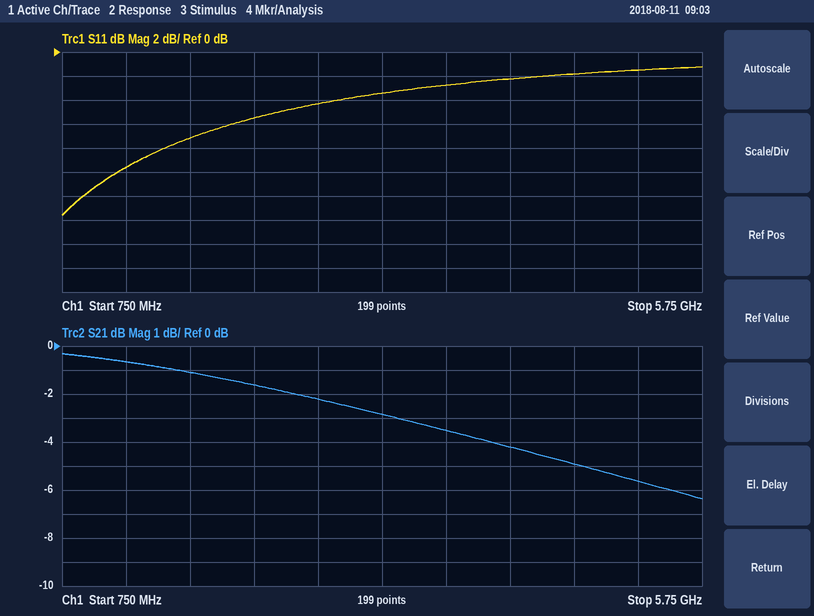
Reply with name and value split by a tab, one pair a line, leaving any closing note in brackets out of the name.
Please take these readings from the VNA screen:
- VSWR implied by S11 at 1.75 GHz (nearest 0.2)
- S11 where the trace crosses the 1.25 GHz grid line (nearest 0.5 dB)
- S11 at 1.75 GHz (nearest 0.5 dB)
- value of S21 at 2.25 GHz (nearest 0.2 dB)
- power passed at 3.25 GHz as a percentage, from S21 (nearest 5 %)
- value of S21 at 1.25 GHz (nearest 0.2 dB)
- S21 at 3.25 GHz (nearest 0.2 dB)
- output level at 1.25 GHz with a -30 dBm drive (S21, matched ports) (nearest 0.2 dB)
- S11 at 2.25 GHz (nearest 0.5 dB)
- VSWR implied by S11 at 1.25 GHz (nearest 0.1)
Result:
VSWR implied by S11 at 1.75 GHz	2.6
S11 where the trace crosses the 1.25 GHz grid line	-9.5 dB
S11 at 1.75 GHz	-7.0 dB
value of S21 at 2.25 GHz	-1.6 dB
power passed at 3.25 GHz as a percentage, from S21	50 %
value of S21 at 1.25 GHz	-0.6 dB
S21 at 3.25 GHz	-2.8 dB
output level at 1.25 GHz with a -30 dBm drive (S21, matched ports)	-30.6 dBm
S11 at 2.25 GHz	-5.5 dB
VSWR implied by S11 at 1.25 GHz	2.0
